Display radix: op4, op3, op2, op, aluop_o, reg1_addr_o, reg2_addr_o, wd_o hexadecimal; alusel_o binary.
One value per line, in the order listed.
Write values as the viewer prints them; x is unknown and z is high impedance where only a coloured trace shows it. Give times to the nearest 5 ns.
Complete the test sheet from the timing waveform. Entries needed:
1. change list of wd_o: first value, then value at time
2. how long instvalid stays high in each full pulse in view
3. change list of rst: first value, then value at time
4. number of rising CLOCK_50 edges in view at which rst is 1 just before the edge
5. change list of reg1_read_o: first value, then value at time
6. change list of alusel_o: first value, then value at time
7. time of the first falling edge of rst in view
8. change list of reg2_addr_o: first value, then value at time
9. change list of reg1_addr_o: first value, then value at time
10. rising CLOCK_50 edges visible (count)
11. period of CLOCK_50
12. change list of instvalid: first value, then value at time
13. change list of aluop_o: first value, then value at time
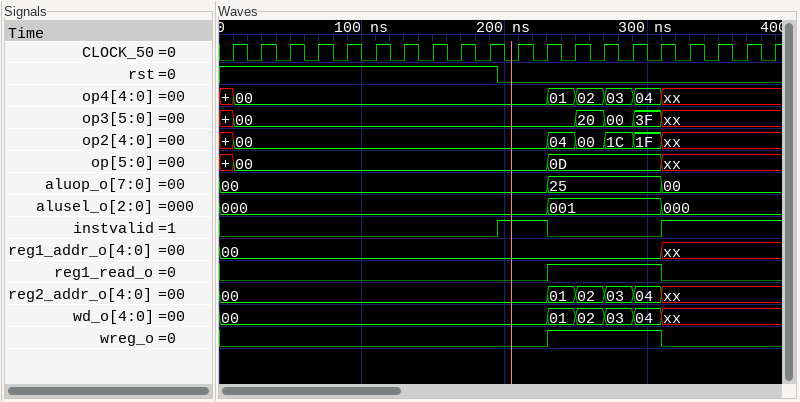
00, 01 at 230 ns, 02 at 250 ns, 03 at 270 ns, 04 at 290 ns, xx at 310 ns
35 ns
1, 0 at 195 ns
10
0, 1 at 230 ns, 0 at 310 ns
000, 001 at 230 ns, 000 at 310 ns
195 ns
00, 01 at 230 ns, 02 at 250 ns, 03 at 270 ns, 04 at 290 ns, xx at 310 ns
00, xx at 310 ns
20
20 ns
0, 1 at 195 ns, 0 at 230 ns, 1 at 310 ns
00, 25 at 230 ns, 00 at 310 ns
